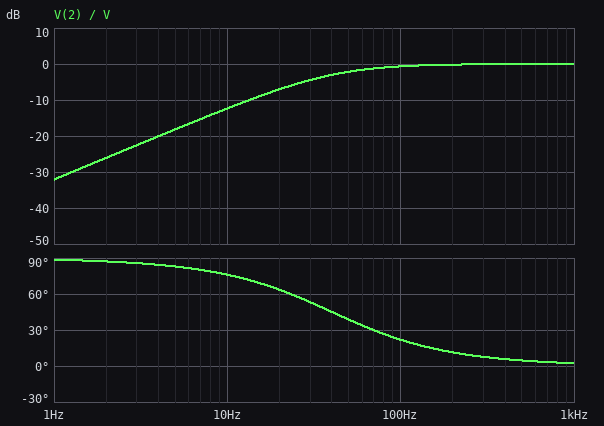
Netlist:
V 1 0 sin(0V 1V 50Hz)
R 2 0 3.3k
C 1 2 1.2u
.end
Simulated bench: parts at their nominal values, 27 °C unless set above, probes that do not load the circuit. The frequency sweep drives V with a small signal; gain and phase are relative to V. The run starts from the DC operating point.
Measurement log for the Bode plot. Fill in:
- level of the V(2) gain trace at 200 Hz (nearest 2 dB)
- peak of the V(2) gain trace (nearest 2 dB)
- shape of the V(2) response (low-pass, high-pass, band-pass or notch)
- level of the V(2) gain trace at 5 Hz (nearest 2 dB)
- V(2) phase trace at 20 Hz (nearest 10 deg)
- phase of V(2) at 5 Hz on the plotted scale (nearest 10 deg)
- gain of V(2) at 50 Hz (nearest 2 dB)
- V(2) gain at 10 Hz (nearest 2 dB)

0 dB
0 dB
high-pass
-18 dB
60 deg
80 deg
-2 dB
-12 dB
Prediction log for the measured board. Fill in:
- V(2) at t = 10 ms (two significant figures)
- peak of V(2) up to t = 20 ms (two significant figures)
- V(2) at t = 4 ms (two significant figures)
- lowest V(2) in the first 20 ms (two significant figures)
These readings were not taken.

-530 mV
560 mV
550 mV
-800 mV
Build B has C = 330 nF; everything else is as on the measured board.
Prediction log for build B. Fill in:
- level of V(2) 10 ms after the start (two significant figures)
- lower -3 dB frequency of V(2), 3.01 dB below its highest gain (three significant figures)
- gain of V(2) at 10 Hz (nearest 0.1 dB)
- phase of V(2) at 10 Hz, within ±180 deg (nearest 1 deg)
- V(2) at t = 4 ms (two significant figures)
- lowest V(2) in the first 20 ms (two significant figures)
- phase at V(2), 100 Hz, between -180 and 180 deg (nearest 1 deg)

-310 mV
146 Hz
-23.3 dB
86 deg
190 mV
-320 mV
56 deg
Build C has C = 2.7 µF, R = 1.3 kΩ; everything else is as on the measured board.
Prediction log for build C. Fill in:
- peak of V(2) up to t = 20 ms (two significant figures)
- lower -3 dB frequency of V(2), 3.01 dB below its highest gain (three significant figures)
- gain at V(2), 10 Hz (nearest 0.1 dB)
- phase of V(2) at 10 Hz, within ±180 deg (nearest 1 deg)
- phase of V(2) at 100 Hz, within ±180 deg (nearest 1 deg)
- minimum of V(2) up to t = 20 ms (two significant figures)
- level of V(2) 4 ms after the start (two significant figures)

530 mV
45.3 Hz
-13.3 dB
78 deg
24 deg
-750 mV
520 mV
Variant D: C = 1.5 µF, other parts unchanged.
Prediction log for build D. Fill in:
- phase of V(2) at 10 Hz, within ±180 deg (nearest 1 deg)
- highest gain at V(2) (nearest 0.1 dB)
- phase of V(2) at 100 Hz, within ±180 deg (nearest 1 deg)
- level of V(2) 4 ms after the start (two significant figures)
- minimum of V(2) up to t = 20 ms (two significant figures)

73 deg
0 dB
18 deg
610 mV
-870 mV
